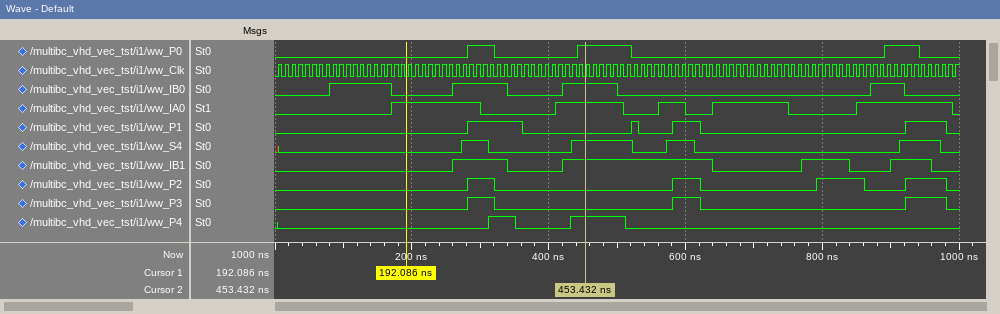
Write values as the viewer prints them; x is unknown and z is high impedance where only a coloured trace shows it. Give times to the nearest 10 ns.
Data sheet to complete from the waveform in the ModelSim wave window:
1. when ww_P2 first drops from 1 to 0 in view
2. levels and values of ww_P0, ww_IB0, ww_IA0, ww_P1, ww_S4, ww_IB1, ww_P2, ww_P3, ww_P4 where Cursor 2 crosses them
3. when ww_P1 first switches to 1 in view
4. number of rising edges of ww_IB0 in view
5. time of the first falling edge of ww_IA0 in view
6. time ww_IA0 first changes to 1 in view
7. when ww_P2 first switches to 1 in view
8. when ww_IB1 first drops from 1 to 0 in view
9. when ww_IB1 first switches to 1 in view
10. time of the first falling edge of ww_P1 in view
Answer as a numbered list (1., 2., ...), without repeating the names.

1. 320 ns
2. ww_P0=1, ww_IB0=1, ww_IA0=1, ww_P1=0, ww_S4=1, ww_IB1=1, ww_P2=0, ww_P3=0, ww_P4=1
3. 280 ns
4. 4
5. 300 ns
6. 170 ns
7. 280 ns
8. 340 ns
9. 260 ns
10. 360 ns
